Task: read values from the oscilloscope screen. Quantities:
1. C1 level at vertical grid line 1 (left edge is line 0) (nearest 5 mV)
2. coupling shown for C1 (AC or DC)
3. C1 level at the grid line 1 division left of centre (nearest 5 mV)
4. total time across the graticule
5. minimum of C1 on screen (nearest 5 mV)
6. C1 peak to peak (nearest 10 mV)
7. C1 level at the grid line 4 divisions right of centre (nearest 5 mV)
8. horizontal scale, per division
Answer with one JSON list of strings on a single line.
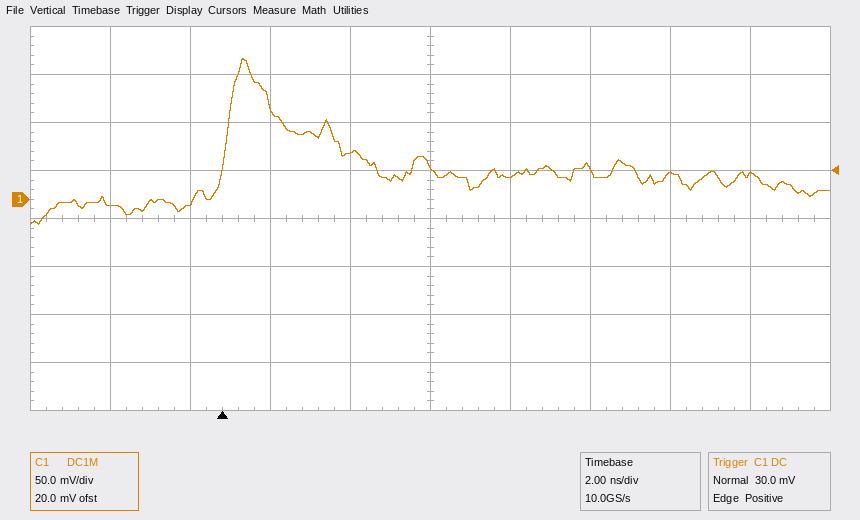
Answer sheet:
["-5 mV", "DC", "50 mV", "20 ns", "-25 mV", "170 mV", "25 mV", "2 ns"]
